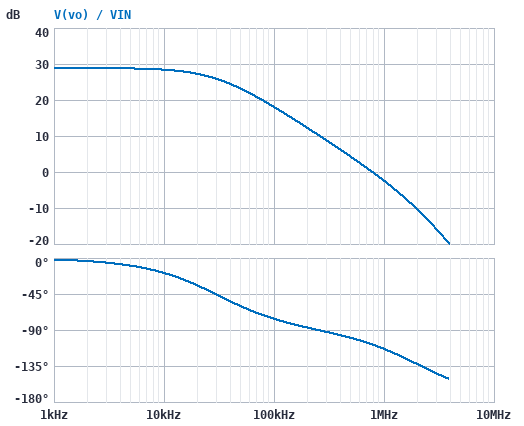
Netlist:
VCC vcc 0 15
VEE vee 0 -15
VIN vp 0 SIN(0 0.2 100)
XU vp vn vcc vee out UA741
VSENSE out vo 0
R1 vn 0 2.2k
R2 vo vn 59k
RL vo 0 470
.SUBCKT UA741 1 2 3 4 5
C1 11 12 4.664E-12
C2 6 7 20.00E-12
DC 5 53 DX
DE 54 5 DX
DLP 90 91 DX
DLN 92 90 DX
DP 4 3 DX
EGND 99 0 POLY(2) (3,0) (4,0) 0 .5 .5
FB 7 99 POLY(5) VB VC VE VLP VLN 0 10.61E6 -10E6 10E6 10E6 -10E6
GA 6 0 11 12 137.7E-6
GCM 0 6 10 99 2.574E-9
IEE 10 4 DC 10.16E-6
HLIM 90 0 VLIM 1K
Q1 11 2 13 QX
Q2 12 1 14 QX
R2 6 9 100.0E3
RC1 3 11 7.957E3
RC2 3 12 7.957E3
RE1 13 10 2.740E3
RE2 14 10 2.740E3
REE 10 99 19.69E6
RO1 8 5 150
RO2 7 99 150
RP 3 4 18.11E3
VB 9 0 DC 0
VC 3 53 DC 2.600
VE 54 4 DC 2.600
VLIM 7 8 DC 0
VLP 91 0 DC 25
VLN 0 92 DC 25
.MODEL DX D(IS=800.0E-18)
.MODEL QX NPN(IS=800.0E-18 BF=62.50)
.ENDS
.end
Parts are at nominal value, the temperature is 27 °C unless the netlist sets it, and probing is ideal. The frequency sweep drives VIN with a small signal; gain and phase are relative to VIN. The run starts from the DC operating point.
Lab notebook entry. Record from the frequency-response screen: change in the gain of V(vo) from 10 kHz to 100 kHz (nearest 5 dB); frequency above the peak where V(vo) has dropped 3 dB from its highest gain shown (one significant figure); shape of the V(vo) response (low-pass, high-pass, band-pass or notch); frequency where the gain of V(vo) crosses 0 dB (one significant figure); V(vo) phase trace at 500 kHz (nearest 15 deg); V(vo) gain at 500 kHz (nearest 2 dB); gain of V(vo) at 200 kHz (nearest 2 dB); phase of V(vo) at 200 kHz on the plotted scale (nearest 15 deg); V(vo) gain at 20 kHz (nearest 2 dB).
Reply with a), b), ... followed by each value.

a) -10 dB
b) 30 kHz
c) low-pass
d) 800 kHz
e) -105 deg
f) 4 dB
g) 12 dB
h) -90 deg
i) 28 dB
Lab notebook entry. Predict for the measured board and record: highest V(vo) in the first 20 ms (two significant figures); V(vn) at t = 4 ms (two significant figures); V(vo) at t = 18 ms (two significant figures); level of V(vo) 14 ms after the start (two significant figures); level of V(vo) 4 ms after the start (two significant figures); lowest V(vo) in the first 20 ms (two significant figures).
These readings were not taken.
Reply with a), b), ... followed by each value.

a) 5.6 V
b) 120 mV
c) -5.3 V
d) 3.3 V
e) 3.3 V
f) -5.6 V
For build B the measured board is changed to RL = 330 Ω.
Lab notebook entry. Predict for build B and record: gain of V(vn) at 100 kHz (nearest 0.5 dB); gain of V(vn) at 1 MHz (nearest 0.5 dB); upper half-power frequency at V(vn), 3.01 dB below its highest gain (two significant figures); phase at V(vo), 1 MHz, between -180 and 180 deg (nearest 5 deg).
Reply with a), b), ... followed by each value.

a) -11.5 dB
b) -32.5 dB
c) 27 kHz
d) -115 deg
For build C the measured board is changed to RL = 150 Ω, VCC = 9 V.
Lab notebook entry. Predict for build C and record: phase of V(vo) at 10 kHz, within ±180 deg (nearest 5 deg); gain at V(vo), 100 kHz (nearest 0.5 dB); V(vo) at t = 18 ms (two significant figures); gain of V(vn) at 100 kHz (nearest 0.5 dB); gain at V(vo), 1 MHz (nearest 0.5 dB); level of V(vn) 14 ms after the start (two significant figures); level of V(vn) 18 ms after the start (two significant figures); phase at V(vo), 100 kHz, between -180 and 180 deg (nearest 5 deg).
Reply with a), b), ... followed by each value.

a) -25 deg
b) 14.5 dB
c) -3.8 V
d) -14.0 dB
e) -6.0 dB
f) 120 mV
g) -140 mV
h) -80 deg
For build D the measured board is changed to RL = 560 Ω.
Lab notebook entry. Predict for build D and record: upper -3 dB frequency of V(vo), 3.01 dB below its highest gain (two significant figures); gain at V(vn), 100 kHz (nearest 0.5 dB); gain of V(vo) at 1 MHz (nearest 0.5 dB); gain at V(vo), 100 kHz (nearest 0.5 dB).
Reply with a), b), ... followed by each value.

a) 31 kHz
b) -10.5 dB
c) -2.0 dB
d) 18.5 dB
